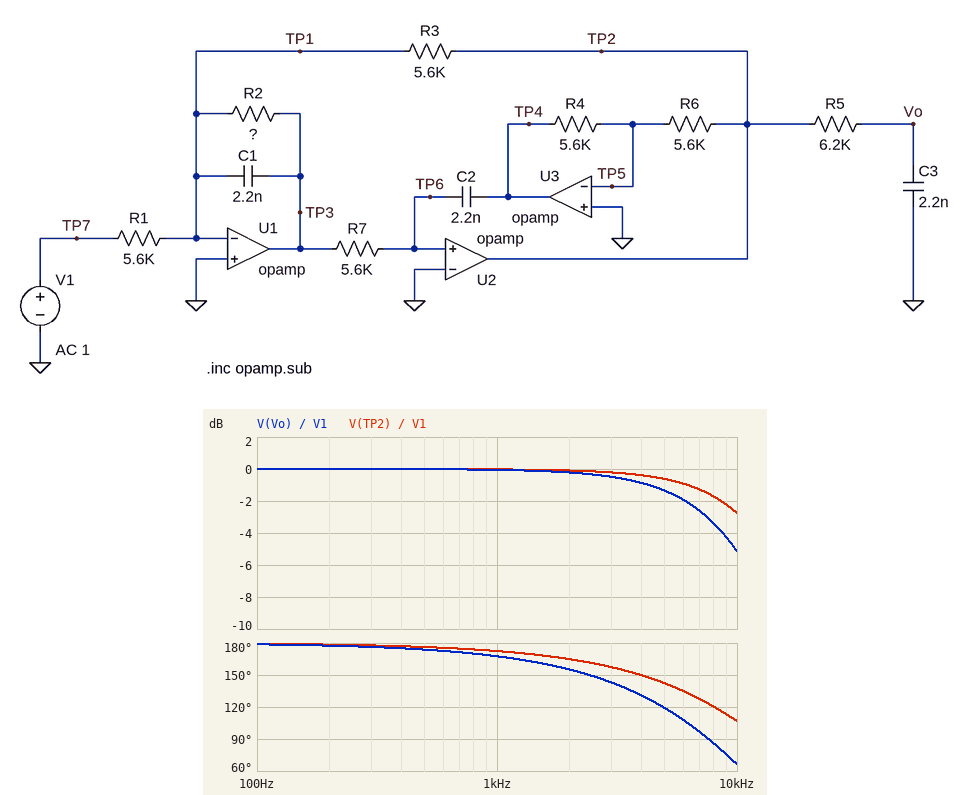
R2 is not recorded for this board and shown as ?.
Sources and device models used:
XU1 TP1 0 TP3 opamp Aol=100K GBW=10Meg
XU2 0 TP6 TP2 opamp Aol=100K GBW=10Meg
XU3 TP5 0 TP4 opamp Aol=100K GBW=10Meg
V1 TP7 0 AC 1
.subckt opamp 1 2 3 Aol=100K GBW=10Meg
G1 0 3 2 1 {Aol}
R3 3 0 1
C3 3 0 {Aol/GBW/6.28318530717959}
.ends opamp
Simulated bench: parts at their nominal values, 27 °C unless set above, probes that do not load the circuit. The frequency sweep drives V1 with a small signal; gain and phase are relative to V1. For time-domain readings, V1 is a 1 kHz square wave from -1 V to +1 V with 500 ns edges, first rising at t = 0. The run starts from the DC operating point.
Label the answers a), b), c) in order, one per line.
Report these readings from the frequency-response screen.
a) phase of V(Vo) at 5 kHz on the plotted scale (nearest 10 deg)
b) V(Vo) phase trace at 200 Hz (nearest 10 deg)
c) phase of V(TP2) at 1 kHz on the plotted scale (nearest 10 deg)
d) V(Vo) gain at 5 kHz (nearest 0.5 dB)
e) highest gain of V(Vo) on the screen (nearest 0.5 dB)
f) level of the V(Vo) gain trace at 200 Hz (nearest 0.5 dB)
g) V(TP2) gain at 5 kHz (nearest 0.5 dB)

a) 120 deg
b) 180 deg
c) 170 deg
d) -1.5 dB
e) 0 dB
f) 0 dB
g) -0.5 dB
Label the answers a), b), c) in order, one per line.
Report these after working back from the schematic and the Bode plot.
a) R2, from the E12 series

a) 3.3 kΩ
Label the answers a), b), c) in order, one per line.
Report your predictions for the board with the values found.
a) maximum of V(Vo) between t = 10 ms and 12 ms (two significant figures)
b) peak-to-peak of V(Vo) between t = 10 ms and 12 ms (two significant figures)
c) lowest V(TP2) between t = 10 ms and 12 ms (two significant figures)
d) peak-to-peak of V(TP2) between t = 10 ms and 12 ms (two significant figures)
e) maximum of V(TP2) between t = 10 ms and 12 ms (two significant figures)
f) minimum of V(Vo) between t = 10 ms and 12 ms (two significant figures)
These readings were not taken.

a) 1.0 V
b) 2.0 V
c) -1.0 V
d) 2.0 V
e) 1.0 V
f) -1.0 V
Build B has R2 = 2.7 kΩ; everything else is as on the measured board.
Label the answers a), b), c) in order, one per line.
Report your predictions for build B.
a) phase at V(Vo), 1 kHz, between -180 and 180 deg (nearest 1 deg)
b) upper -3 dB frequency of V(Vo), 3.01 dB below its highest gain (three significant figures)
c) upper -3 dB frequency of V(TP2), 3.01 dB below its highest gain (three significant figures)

a) 166 deg
b) 6.12 kHz
c) 7.89 kHz
